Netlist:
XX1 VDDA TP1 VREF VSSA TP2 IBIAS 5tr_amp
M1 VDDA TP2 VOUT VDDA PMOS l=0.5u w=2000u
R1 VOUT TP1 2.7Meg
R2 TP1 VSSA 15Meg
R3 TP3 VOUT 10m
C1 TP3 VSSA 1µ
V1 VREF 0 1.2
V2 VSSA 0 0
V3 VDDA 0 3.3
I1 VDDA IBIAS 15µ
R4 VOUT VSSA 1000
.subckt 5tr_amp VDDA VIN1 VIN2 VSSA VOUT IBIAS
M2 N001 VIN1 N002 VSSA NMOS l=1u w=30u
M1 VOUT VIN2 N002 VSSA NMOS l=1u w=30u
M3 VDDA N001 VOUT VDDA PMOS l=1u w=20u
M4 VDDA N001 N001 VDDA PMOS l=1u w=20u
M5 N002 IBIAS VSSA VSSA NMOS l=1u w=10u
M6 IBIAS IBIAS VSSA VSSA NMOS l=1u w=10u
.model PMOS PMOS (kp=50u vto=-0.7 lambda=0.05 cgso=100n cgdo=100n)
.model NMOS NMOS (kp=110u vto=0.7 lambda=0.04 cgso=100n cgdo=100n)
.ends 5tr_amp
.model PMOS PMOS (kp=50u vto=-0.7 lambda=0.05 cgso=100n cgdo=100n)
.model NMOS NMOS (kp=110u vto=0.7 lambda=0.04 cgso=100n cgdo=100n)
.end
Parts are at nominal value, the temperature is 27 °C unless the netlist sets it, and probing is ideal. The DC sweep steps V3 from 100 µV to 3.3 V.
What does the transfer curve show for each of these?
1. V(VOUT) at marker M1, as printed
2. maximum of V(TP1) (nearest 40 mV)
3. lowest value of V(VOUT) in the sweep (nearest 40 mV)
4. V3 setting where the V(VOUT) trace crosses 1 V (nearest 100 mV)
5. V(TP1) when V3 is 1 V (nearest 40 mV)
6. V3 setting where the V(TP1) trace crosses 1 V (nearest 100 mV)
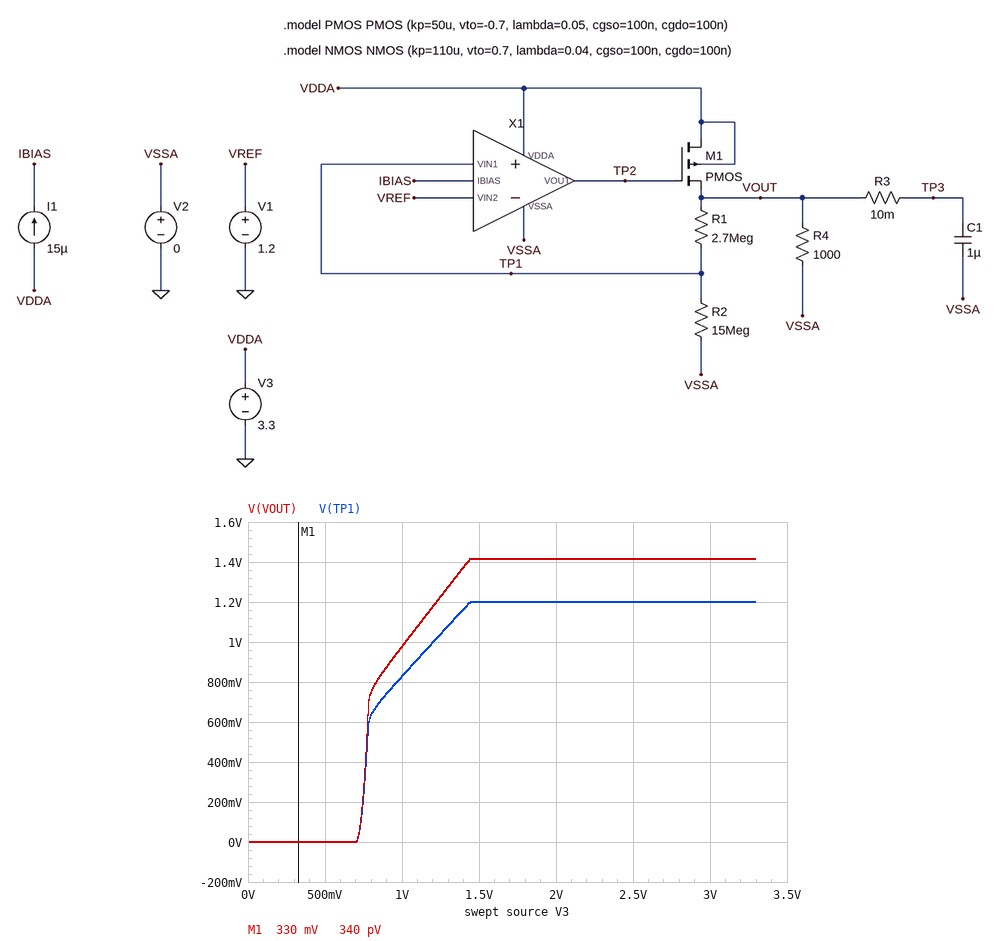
340 pV
1.20 V
0 V
1.0 V
840 mV
1.2 V
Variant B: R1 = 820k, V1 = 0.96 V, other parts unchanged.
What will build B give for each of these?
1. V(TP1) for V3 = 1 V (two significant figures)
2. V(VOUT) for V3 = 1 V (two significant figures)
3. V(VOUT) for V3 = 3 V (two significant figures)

910 mV
960 mV
1.0 V
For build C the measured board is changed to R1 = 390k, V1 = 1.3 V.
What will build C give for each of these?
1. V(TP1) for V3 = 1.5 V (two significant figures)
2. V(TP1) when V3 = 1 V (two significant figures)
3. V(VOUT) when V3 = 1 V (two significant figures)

1.3 V
940 mV
960 mV
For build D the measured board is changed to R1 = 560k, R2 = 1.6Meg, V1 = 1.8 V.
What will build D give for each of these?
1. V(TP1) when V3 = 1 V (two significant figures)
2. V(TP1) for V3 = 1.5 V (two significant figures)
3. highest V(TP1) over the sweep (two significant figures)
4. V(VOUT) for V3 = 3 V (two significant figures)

730 mV
1.1 V
1.8 V
2.4 V
